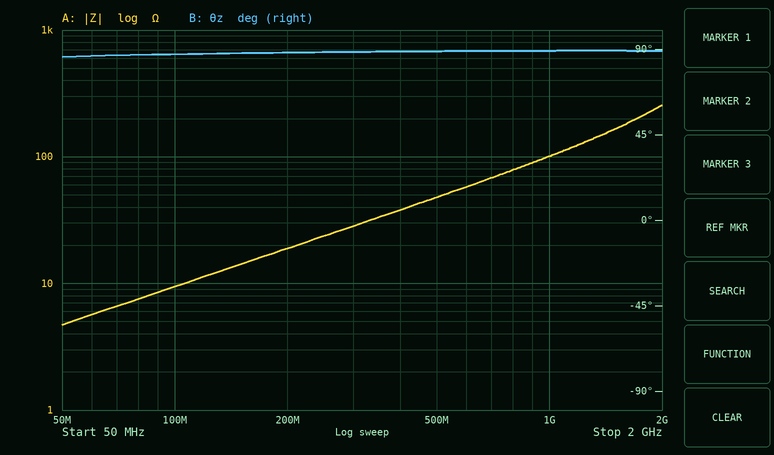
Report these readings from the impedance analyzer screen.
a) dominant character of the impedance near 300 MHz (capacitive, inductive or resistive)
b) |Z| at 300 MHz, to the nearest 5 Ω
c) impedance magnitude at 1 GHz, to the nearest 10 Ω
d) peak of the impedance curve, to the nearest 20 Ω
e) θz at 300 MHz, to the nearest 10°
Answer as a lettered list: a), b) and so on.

a) inductive
b) 30 Ω
c) 100 Ω
d) 260 Ω
e) 90°
